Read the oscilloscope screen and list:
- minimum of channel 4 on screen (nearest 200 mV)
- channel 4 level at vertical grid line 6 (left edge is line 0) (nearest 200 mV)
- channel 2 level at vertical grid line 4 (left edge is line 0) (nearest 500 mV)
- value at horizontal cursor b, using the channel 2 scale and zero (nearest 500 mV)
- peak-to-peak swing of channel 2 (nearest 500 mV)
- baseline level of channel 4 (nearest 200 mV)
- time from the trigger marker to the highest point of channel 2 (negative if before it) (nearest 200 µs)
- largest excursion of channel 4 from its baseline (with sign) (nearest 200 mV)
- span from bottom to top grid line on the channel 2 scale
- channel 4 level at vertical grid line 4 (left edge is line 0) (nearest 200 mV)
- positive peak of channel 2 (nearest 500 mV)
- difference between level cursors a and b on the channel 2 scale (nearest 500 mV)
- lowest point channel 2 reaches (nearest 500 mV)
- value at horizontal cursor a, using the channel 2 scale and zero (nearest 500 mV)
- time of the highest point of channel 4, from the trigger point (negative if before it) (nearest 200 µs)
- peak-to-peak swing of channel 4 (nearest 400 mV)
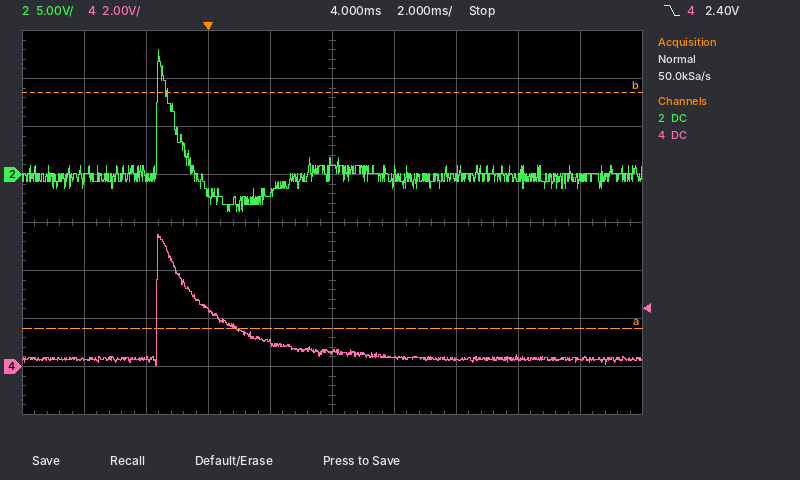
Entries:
0.0 V
400 mV
-2.0 V
8.5 V
17.0 V
400 mV
-1.6 ms
+5.2 V
40 V
1.0 V
13.0 V
24.5 V
-4.0 V
-16.0 V
-1.6 ms
5.6 V
